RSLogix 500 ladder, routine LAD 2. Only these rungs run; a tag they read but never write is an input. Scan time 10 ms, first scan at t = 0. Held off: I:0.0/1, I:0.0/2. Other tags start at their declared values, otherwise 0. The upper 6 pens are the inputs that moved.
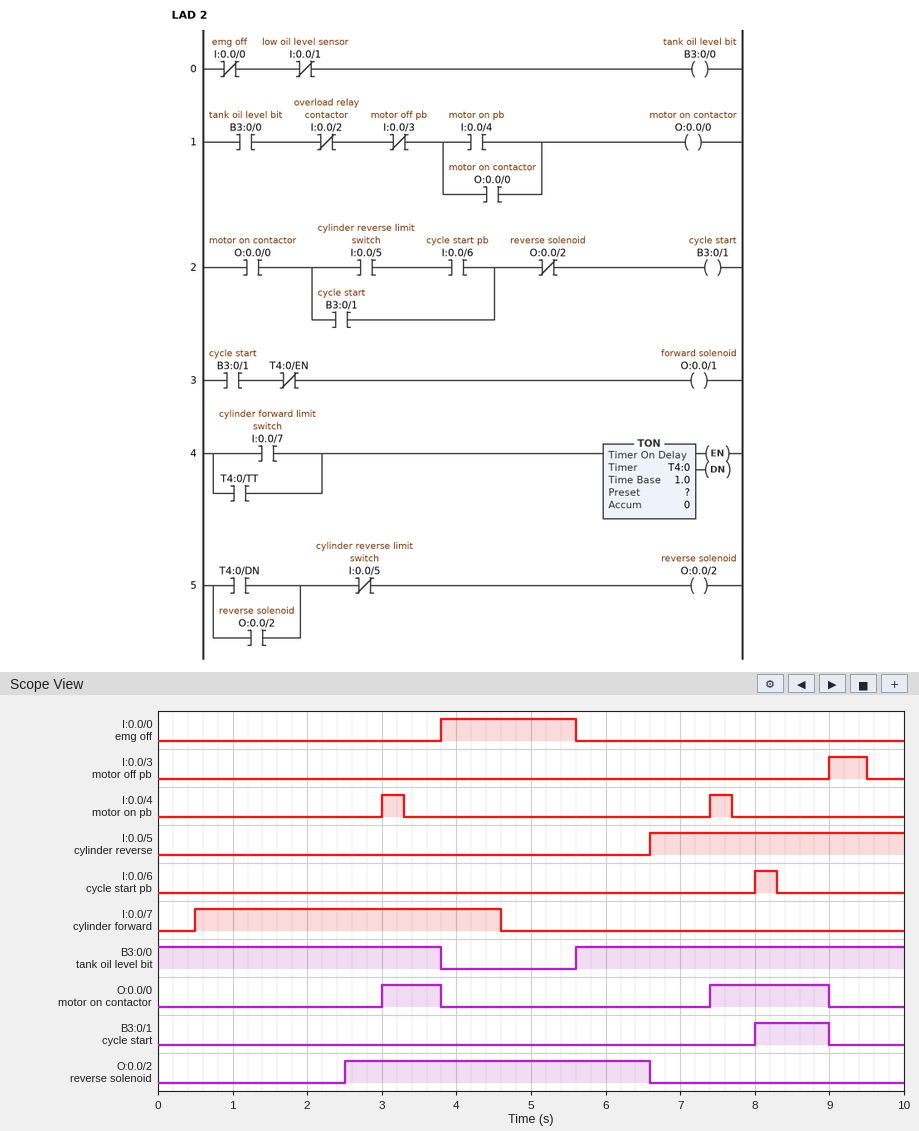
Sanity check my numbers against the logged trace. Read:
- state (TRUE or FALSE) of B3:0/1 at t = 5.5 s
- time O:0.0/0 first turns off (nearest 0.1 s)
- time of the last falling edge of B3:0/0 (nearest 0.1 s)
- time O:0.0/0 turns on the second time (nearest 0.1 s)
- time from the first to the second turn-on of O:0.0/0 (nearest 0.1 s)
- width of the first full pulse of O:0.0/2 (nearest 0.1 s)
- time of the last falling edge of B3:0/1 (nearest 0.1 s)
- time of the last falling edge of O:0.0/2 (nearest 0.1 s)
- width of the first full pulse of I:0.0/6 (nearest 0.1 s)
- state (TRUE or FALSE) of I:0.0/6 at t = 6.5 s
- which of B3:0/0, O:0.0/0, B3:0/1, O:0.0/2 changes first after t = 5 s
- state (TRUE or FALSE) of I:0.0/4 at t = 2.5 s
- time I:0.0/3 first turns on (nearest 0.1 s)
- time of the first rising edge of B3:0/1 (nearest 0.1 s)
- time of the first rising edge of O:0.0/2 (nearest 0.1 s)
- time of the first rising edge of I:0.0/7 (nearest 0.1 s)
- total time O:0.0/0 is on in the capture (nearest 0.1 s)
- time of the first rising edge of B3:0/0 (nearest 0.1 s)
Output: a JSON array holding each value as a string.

["FALSE", "3.8 s", "3.8 s", "7.4 s", "4.4 s", "4.1 s", "9.0 s", "6.6 s", "0.3 s", "FALSE", "B3:0/0", "FALSE", "9.0 s", "8.0 s", "2.5 s", "0.5 s", "2.4 s", "5.6 s"]
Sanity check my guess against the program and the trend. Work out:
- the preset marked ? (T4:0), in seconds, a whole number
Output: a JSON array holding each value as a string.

["2 s"]
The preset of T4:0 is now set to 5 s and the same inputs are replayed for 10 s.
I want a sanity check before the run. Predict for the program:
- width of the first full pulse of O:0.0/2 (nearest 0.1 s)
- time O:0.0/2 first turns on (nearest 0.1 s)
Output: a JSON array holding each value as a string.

["1.1 s", "5.5 s"]
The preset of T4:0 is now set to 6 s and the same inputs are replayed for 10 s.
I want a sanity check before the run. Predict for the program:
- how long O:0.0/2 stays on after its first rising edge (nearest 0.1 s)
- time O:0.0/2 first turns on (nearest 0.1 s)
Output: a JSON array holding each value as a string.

["0.1 s", "6.5 s"]
